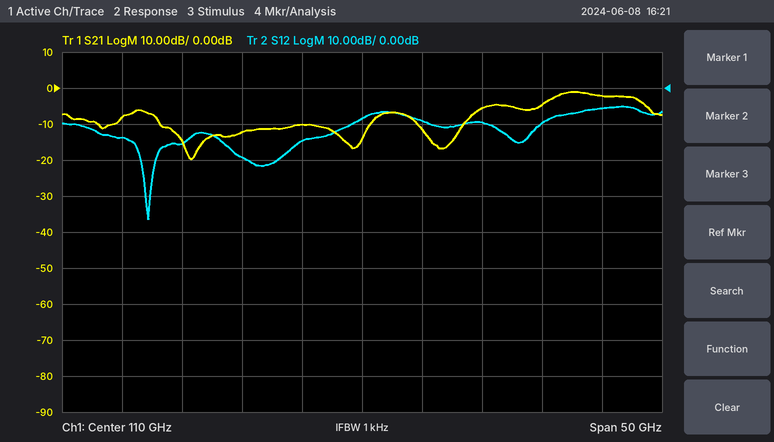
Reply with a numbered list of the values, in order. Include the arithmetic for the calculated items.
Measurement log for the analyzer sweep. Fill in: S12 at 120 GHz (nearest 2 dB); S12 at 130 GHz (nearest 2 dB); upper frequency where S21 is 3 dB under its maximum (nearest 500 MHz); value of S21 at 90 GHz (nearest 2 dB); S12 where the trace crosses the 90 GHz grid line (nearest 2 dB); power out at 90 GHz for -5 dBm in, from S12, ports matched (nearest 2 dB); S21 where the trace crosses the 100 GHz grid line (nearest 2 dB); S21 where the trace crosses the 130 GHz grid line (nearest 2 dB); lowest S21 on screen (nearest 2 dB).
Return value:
1. -10 dB
2. -6 dB
3. 133.5 GHz
4. -8 dB
5. -14 dB
6. -5 dBm + (-14 dB) = -18 dBm
7. -12 dB
8. -2 dB
9. -20 dB
